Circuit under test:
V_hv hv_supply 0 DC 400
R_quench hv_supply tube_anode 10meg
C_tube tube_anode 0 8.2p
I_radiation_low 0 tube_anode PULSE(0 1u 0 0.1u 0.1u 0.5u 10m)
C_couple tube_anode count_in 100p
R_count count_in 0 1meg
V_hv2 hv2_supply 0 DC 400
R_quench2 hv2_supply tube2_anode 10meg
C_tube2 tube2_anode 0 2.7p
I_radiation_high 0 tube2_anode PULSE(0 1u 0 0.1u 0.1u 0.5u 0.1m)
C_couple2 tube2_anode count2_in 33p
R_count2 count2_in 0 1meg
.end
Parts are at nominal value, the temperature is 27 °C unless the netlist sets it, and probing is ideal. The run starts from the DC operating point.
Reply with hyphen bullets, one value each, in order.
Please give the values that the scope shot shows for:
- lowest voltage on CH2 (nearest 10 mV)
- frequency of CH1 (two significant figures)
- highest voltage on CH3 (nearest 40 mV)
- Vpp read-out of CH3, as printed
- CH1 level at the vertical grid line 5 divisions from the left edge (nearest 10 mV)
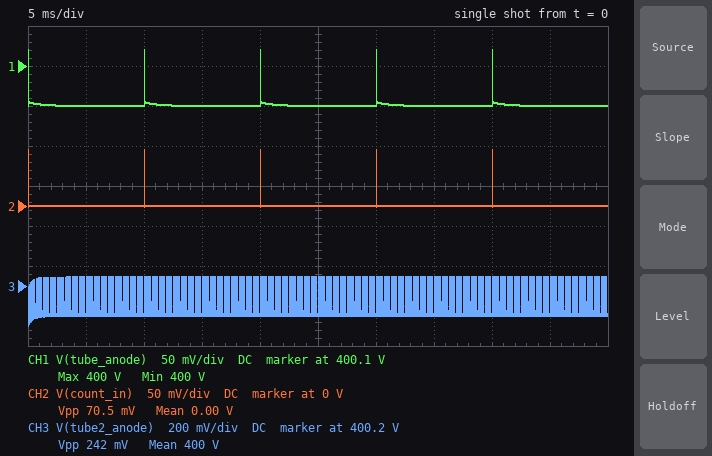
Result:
- 0 V
- 100 Hz
- 400.24 V
- 242 mV
- 400.00 V
